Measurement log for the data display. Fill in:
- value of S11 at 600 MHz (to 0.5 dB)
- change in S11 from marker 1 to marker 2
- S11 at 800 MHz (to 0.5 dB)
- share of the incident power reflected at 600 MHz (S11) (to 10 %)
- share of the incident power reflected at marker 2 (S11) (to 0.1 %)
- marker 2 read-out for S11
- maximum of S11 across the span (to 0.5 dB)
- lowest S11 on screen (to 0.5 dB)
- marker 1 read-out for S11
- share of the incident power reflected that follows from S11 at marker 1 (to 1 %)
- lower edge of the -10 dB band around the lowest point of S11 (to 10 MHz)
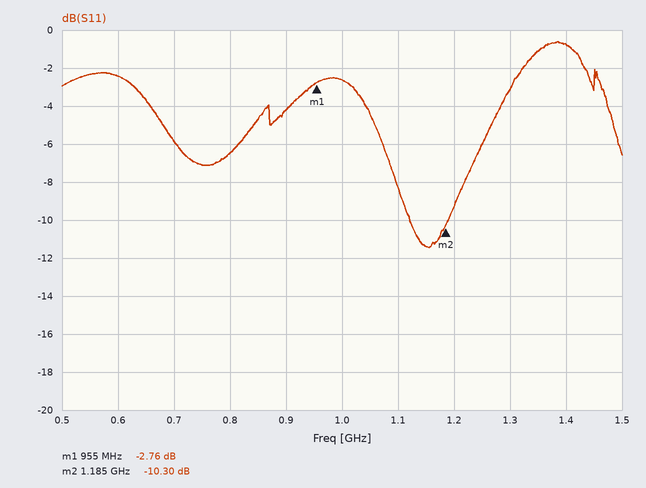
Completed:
-2.5 dB
-7.54 dB
-6.5 dB
60 %
9.3 %
-10.30 dB
-0.5 dB
-11.5 dB
-2.76 dB
53 %
1.12 GHz
